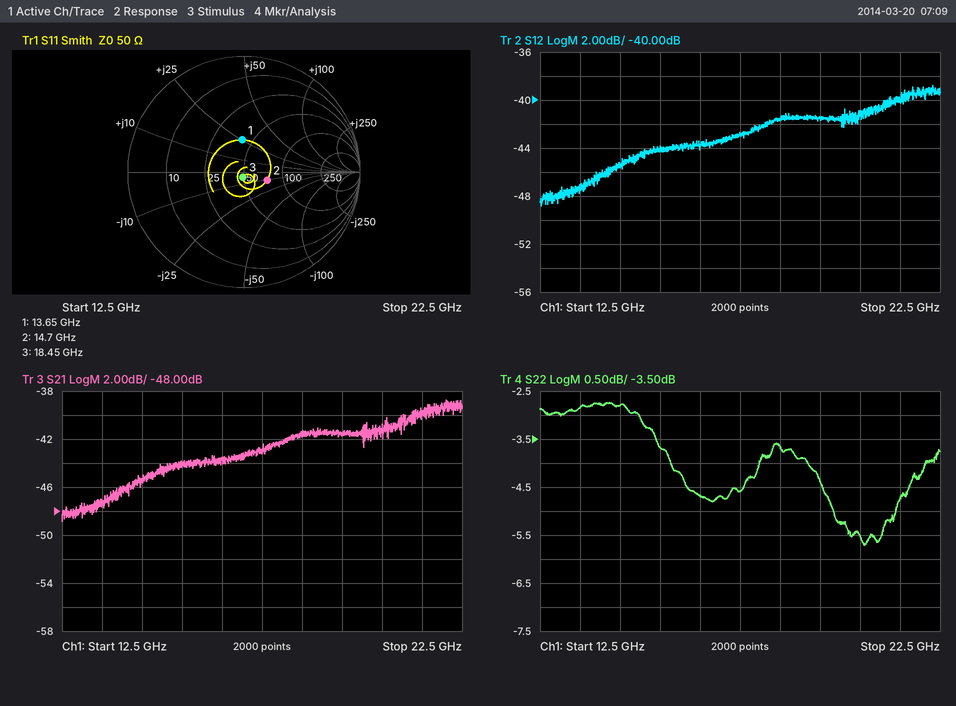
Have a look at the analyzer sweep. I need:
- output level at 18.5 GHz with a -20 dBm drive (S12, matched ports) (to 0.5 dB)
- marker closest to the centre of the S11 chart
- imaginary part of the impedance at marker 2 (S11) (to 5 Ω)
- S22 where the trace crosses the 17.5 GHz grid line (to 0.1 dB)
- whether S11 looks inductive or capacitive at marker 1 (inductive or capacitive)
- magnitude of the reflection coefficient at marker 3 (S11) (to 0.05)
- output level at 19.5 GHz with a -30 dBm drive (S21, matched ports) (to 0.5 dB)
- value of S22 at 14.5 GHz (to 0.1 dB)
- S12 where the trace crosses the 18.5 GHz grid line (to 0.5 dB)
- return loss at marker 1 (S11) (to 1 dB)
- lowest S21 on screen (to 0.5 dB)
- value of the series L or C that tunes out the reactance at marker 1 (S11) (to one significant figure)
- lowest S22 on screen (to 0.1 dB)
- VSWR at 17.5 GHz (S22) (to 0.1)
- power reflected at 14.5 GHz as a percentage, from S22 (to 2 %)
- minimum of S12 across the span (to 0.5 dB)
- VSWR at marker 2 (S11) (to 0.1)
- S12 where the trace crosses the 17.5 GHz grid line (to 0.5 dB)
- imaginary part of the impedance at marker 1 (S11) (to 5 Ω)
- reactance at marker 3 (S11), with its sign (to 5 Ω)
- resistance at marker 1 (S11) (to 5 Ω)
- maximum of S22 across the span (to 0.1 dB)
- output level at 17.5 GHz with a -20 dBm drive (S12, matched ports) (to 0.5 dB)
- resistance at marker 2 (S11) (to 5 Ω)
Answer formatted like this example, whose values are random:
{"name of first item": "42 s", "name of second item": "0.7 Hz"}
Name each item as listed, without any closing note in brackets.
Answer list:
{"output level at 18.5 GHz with a -20 dBm drive (S12, matched ports)": "-61.5 dBm", "marker closest to the centre of the S11 chart": "marker 3", "imaginary part of the impedance at marker 2 (S11)": "-10 Ω", "S22 where the trace crosses the 17.5 GHz grid line": "-4.6 dB", "whether S11 looks inductive or capacitive at marker 1": "inductive", "magnitude of the reflection coefficient at marker 3 (S11)": "0.05", "output level at 19.5 GHz with a -30 dBm drive (S21, matched ports)": "-71.5 dBm", "value of S22 at 14.5 GHz": "-2.8 dB", "S12 where the trace crosses the 18.5 GHz grid line": "-41.5 dB", "return loss at marker 1 (S11)": "11 dB", "lowest S21 on screen": "-49.0 dB", "value of the series L or C that tunes out the reactance at marker 1 (S11)": "500 fF", "lowest S22 on screen": "-5.7 dB", "VSWR at 17.5 GHz (S22)": "3.9", "power reflected at 14.5 GHz as a percentage, from S22": "52 %", "minimum of S12 across the span": "-49.0 dB", "VSWR at marker 2 (S11)": "1.5", "S12 where the trace crosses the 17.5 GHz grid line": "-43.0 dB", "imaginary part of the impedance at marker 1 (S11)": "+25 Ω", "reactance at marker 3 (S11), with its sign": "-5 Ω", "resistance at marker 1 (S11)": "40 Ω", "maximum of S22 across the span": "-2.7 dB", "output level at 17.5 GHz with a -20 dBm drive (S12, matched ports)": "-63.0 dBm", "resistance at marker 2 (S11)": "75 Ω"}
